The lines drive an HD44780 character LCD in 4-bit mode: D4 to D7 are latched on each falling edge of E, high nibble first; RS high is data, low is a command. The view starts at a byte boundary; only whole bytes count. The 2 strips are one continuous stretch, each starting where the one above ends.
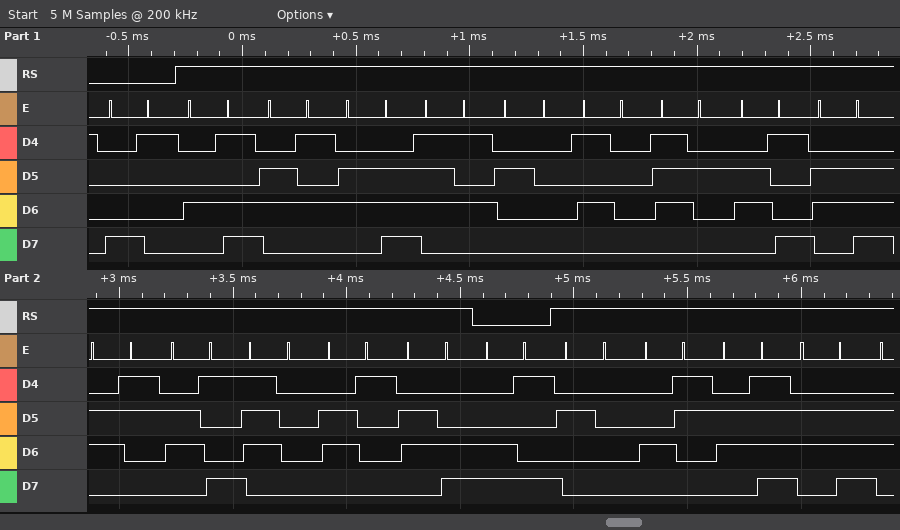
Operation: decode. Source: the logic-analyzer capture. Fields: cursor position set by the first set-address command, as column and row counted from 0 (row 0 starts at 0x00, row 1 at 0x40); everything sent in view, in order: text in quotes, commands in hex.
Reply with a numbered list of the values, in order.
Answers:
1. column 1, row 0
2. 0x81 "Menu Principal" 0xC9 " Con"
